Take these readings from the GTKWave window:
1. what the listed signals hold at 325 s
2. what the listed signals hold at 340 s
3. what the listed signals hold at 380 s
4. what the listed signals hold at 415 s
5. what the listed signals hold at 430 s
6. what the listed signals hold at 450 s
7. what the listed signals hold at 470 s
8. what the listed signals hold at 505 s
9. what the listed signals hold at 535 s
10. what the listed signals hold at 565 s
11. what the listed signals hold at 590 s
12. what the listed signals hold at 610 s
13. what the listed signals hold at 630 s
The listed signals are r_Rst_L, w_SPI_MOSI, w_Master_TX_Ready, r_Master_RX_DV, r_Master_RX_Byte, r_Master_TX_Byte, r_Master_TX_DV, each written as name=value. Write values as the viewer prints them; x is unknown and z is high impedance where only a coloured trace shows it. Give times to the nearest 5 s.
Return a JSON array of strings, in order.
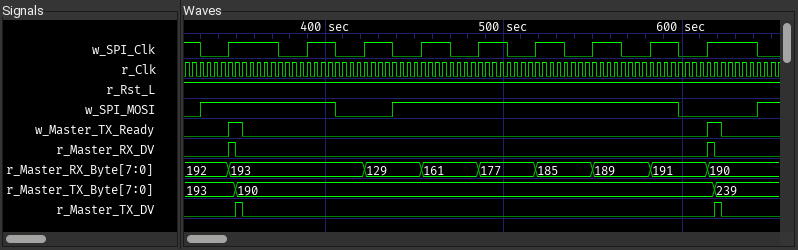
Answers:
["r_Rst_L=1, w_SPI_MOSI=0, w_Master_TX_Ready=0, r_Master_RX_DV=0, r_Master_RX_Byte=192, r_Master_TX_Byte=193, r_Master_TX_DV=0", "r_Rst_L=1, w_SPI_MOSI=1, w_Master_TX_Ready=0, r_Master_RX_DV=0, r_Master_RX_Byte=192, r_Master_TX_Byte=193, r_Master_TX_DV=0", "r_Rst_L=1, w_SPI_MOSI=1, w_Master_TX_Ready=0, r_Master_RX_DV=0, r_Master_RX_Byte=193, r_Master_TX_Byte=190, r_Master_TX_DV=0", "r_Rst_L=1, w_SPI_MOSI=0, w_Master_TX_Ready=0, r_Master_RX_DV=0, r_Master_RX_Byte=193, r_Master_TX_Byte=190, r_Master_TX_DV=0", "r_Rst_L=1, w_SPI_MOSI=0, w_Master_TX_Ready=0, r_Master_RX_DV=0, r_Master_RX_Byte=129, r_Master_TX_Byte=190, r_Master_TX_DV=0", "r_Rst_L=1, w_SPI_MOSI=1, w_Master_TX_Ready=0, r_Master_RX_DV=0, r_Master_RX_Byte=129, r_Master_TX_Byte=190, r_Master_TX_DV=0", "r_Rst_L=1, w_SPI_MOSI=1, w_Master_TX_Ready=0, r_Master_RX_DV=0, r_Master_RX_Byte=161, r_Master_TX_Byte=190, r_Master_TX_DV=0", "r_Rst_L=1, w_SPI_MOSI=1, w_Master_TX_Ready=0, r_Master_RX_DV=0, r_Master_RX_Byte=177, r_Master_TX_Byte=190, r_Master_TX_DV=0", "r_Rst_L=1, w_SPI_MOSI=1, w_Master_TX_Ready=0, r_Master_RX_DV=0, r_Master_RX_Byte=185, r_Master_TX_Byte=190, r_Master_TX_DV=0", "r_Rst_L=1, w_SPI_MOSI=1, w_Master_TX_Ready=0, r_Master_RX_DV=0, r_Master_RX_Byte=189, r_Master_TX_Byte=190, r_Master_TX_DV=0", "r_Rst_L=1, w_SPI_MOSI=1, w_Master_TX_Ready=0, r_Master_RX_DV=0, r_Master_RX_Byte=191, r_Master_TX_Byte=190, r_Master_TX_DV=0", "r_Rst_L=1, w_SPI_MOSI=0, w_Master_TX_Ready=0, r_Master_RX_DV=0, r_Master_RX_Byte=191, r_Master_TX_Byte=190, r_Master_TX_DV=0", "r_Rst_L=1, w_SPI_MOSI=0, w_Master_TX_Ready=0, r_Master_RX_DV=0, r_Master_RX_Byte=190, r_Master_TX_Byte=239, r_Master_TX_DV=0"]
